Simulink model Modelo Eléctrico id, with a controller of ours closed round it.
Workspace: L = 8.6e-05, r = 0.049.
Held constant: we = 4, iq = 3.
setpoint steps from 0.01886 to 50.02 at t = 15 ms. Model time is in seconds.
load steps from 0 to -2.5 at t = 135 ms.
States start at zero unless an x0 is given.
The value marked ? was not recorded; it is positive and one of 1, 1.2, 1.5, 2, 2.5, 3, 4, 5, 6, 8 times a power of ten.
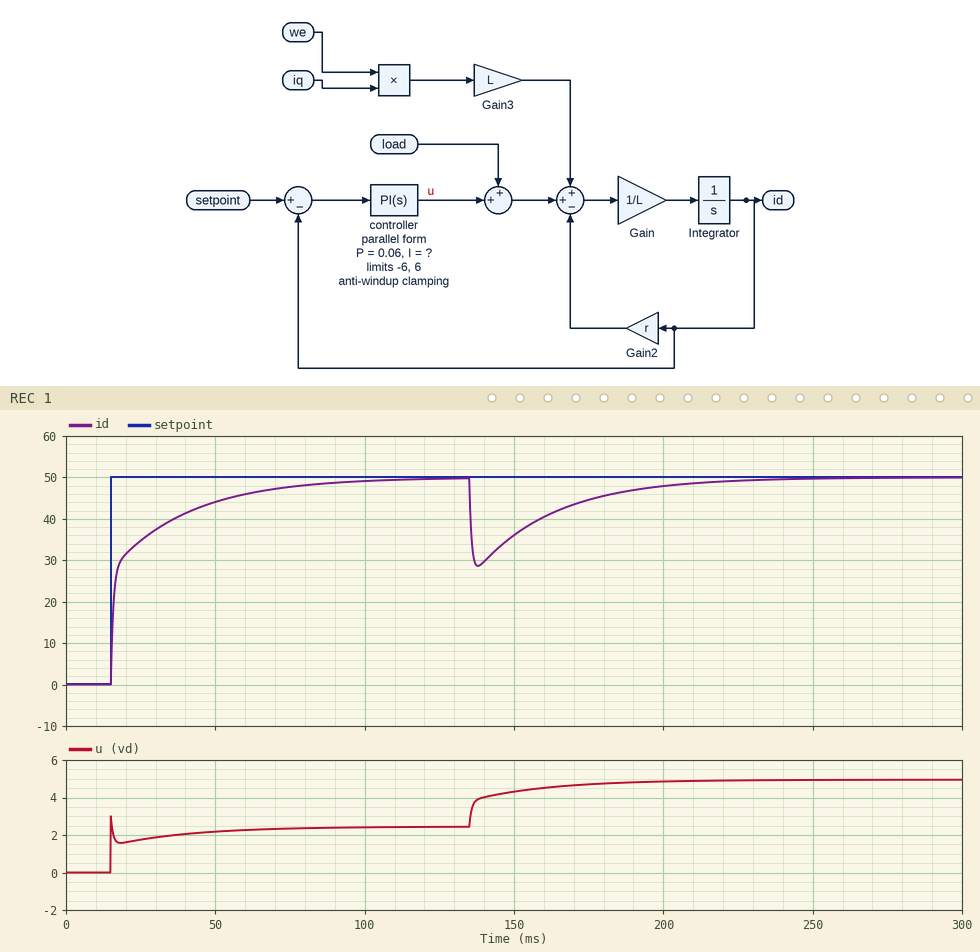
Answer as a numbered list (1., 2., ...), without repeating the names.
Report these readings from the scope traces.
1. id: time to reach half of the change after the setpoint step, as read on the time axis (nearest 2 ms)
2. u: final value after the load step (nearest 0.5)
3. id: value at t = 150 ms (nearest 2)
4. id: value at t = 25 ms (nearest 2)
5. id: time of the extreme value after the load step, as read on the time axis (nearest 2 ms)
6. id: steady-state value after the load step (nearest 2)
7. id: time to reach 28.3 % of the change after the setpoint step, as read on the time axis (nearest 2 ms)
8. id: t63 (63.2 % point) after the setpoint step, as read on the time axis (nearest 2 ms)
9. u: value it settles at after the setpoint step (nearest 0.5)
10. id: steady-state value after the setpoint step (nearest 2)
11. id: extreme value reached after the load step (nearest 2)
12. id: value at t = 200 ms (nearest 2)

1. 16 ms
2. 5.0
3. 36
4. 34
5. 138 ms
6. 50
7. 16 ms
8. 20 ms
9. 2.5
10. 50
11. 28
12. 48
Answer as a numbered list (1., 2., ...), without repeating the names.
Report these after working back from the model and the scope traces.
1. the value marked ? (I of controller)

1. 4
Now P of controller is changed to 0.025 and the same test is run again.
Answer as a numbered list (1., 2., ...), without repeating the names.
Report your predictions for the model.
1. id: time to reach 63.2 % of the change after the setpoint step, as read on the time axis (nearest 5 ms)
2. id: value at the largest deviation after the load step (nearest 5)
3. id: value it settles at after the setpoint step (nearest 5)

1. 25 ms
2. 20
3. 50
